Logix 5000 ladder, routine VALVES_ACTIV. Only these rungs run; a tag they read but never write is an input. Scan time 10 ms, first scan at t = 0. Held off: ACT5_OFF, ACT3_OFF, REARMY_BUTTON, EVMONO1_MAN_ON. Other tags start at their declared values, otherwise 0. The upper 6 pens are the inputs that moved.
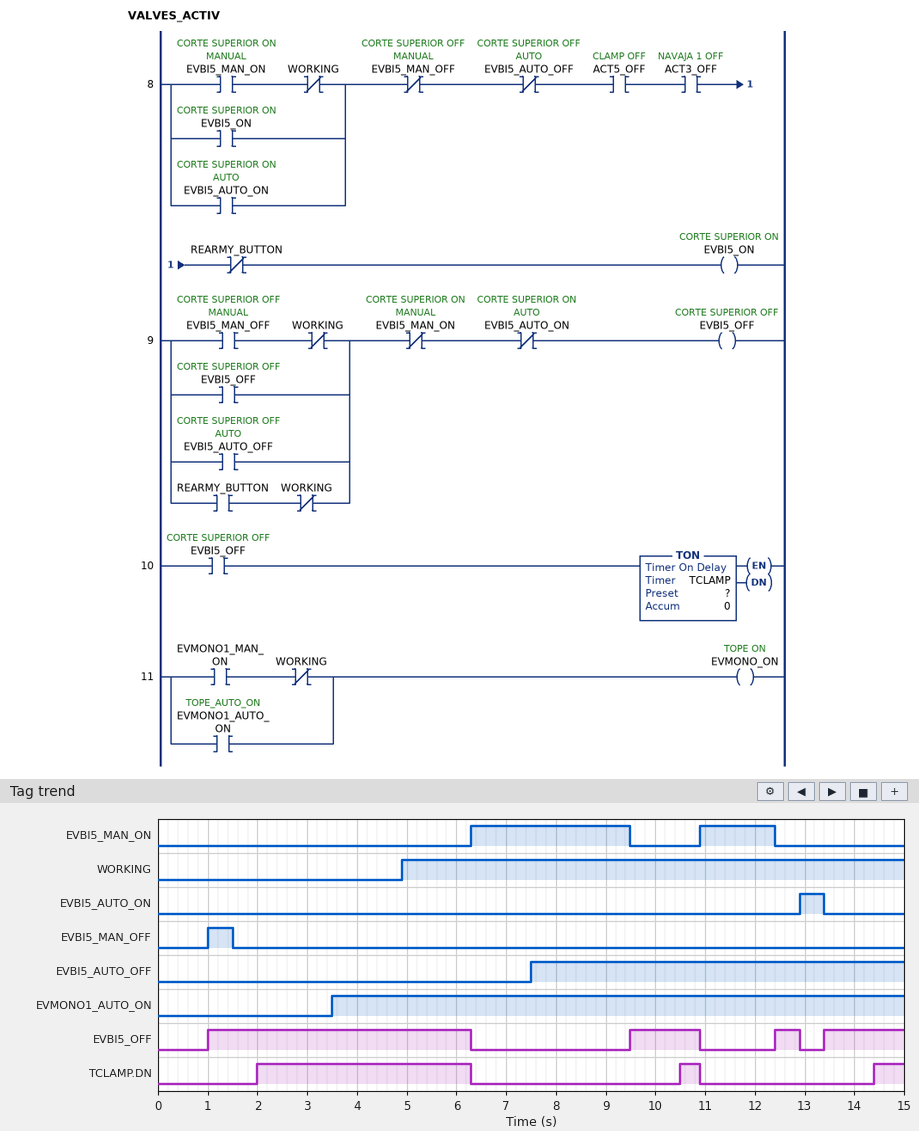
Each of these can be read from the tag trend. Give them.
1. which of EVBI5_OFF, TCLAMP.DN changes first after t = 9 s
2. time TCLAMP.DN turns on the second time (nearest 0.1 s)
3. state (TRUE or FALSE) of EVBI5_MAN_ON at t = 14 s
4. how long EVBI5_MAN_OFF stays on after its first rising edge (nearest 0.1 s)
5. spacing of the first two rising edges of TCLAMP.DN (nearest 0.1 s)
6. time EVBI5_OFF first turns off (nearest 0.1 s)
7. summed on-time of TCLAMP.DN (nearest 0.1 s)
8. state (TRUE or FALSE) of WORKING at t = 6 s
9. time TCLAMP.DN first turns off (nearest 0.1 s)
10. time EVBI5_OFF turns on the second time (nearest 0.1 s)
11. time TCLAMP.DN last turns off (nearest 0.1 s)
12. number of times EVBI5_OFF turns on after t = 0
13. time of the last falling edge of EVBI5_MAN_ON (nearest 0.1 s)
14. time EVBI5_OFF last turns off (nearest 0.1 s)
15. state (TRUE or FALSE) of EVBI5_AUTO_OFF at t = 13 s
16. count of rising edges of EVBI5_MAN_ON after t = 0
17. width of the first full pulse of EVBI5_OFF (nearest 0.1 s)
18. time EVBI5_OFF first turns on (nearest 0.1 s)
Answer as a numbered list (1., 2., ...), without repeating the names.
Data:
1. EVBI5_OFF
2. 10.5 s
3. FALSE
4. 0.5 s
5. 8.5 s
6. 6.3 s
7. 5.3 s
8. TRUE
9. 6.3 s
10. 9.5 s
11. 10.9 s
12. 4
13. 12.4 s
14. 12.9 s
15. TRUE
16. 2
17. 5.3 s
18. 1.0 s
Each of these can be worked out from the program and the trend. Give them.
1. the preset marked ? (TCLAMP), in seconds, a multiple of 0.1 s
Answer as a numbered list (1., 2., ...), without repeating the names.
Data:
1. 1.0 s
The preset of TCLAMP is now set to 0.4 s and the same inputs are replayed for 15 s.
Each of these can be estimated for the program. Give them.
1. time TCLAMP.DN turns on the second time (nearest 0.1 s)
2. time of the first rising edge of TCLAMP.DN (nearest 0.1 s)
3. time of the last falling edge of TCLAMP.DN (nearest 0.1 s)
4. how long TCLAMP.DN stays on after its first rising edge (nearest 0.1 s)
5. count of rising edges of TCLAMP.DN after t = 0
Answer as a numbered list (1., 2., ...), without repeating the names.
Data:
1. 9.9 s
2. 1.4 s
3. 12.9 s
4. 4.9 s
5. 4
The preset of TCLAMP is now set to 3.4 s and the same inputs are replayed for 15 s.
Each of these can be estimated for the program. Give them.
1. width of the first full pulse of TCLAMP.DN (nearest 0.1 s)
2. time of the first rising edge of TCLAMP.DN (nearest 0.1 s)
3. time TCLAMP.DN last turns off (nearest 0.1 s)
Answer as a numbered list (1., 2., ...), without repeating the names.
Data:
1. 1.9 s
2. 4.4 s
3. 6.3 s
